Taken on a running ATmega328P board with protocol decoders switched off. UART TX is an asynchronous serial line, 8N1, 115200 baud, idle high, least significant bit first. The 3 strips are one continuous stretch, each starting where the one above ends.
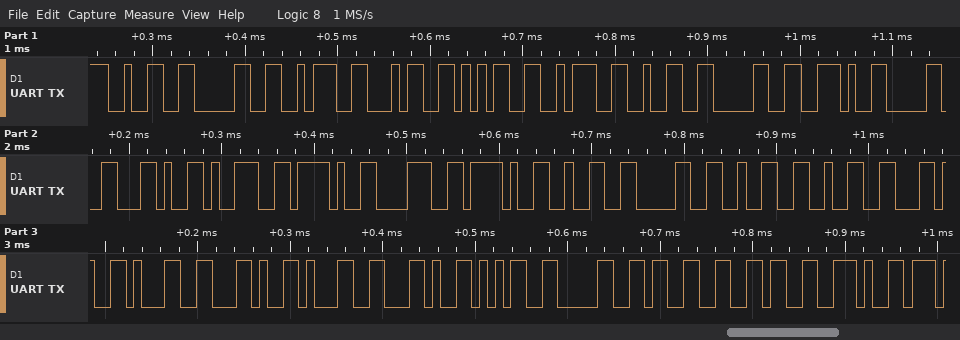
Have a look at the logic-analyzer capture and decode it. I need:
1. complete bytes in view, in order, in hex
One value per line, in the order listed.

32 30 3A 34 35 3A 32 30 2E 30 2C 39 2F 38 2F 32 30 32 32 2C 31 2C 31 2C 35 30 33 36 2E
